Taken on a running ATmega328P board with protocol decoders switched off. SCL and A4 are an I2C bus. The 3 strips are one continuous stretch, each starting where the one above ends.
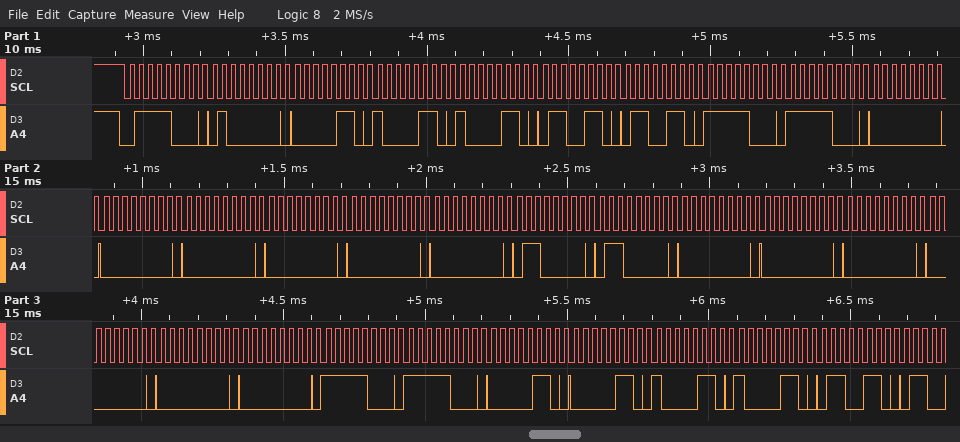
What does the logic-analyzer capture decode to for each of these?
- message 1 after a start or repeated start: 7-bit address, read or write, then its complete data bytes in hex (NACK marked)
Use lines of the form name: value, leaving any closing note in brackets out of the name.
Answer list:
message 1 after a start or repeated start: 7-bit address, read or write, then its complete data bytes in hex: 0x3C write: 40 06 86 86 66 66 F8 F8 00 00 00 00 00 00 60 60 00 00 00 00 00 00 F8 F8 06 06 86 86 66
